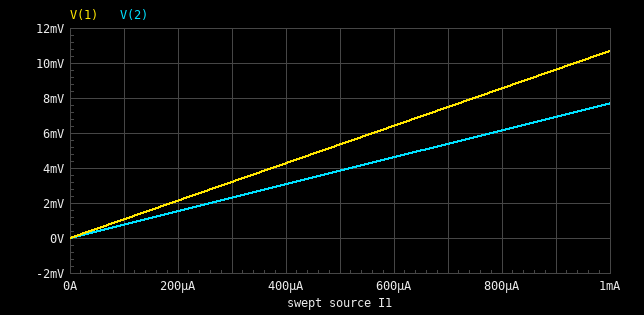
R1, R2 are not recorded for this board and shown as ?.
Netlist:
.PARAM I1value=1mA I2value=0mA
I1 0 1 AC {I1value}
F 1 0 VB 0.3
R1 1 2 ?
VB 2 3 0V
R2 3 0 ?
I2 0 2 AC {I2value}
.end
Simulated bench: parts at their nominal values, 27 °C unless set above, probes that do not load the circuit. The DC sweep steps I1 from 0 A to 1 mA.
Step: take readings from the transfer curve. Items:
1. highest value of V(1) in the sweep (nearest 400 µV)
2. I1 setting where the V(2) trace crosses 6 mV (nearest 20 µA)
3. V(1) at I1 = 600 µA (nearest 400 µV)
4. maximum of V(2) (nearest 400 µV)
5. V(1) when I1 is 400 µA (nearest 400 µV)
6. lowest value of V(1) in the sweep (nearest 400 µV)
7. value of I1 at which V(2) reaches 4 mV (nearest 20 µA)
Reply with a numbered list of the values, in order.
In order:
1. 10.8 mV
2. 780 µA
3. 6.4 mV
4. 7.6 mV
5. 4.4 mV
6. 0 V
7. 520 µA
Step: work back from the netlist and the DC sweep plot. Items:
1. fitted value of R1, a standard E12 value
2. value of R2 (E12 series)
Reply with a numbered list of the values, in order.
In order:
1. 3.9 Ω
2. 10 Ω
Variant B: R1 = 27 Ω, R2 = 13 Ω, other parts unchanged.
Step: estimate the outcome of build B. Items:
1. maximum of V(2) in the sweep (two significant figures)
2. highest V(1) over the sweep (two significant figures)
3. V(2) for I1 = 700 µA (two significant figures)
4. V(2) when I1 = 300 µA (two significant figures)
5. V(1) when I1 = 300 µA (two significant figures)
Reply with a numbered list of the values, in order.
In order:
1. 10 mV
2. 31 mV
3. 7.0 mV
4. 3.0 mV
5. 9.2 mV
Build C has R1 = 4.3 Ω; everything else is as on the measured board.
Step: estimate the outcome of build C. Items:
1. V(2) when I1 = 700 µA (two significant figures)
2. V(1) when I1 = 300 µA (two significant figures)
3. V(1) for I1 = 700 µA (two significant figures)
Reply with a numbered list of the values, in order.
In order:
1. 5.4 mV
2. 3.3 mV
3. 7.7 mV
